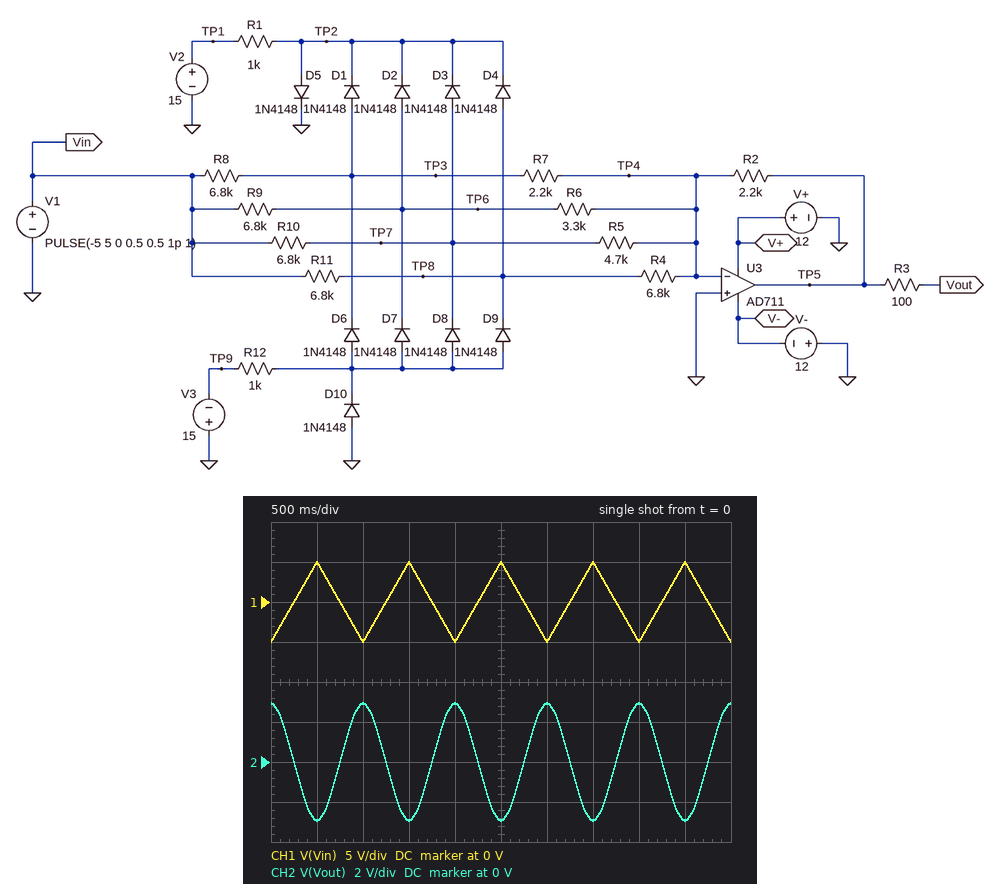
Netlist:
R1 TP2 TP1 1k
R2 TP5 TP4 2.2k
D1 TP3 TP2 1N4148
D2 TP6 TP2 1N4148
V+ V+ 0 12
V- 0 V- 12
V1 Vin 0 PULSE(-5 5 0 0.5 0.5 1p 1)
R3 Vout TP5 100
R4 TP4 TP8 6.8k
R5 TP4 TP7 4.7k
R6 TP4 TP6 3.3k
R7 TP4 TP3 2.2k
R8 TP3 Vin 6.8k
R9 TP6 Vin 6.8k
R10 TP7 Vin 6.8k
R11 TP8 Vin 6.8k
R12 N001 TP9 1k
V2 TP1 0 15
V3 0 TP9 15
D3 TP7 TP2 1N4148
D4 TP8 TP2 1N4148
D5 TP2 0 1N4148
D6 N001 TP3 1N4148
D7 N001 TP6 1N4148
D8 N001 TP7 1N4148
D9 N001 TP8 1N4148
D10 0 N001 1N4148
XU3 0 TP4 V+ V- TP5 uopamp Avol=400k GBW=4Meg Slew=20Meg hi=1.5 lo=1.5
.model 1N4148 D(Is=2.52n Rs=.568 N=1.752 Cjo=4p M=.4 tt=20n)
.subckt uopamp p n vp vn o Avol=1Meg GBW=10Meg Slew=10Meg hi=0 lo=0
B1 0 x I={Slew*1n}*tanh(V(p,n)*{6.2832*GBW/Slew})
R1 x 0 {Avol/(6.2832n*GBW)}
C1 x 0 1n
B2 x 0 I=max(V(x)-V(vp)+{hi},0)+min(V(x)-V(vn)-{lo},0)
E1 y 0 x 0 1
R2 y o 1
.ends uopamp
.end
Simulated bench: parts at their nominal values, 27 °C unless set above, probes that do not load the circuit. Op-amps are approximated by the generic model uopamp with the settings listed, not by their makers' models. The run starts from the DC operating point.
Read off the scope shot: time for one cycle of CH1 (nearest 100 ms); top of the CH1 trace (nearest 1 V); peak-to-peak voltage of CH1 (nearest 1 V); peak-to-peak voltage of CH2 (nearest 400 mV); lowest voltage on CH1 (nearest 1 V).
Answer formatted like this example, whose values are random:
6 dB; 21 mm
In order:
1.0 s; 5 V; 10 V; 6.0 V; -5 V
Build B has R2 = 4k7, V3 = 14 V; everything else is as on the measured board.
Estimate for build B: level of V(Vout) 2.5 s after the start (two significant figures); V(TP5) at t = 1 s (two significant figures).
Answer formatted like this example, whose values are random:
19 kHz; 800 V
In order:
-6.3 V; 6.3 V
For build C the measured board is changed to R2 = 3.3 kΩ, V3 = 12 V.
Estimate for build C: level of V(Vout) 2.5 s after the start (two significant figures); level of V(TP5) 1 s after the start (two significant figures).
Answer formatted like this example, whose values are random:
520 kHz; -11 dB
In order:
-4.4 V; 4.4 V
